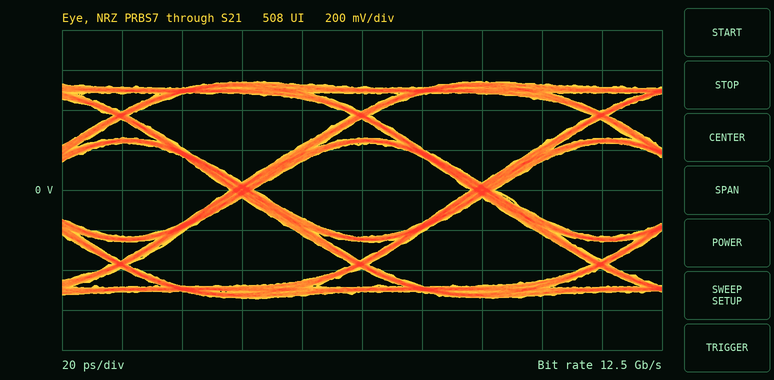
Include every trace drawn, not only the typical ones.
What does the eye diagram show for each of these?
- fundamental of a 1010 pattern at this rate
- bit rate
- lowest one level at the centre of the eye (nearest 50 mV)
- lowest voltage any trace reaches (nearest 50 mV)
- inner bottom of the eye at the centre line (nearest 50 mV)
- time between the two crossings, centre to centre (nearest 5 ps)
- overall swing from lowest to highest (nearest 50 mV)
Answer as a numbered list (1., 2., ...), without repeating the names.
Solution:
1. 6.25 GHz
2. 12.5 Gb/s
3. 250 mV
4. -550 mV
5. -250 mV
6. 80 ps
7. 1.10 V
